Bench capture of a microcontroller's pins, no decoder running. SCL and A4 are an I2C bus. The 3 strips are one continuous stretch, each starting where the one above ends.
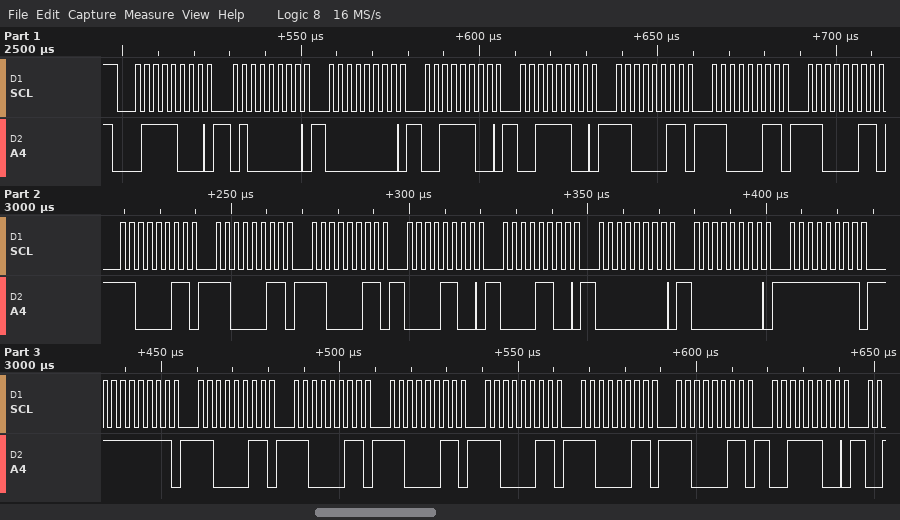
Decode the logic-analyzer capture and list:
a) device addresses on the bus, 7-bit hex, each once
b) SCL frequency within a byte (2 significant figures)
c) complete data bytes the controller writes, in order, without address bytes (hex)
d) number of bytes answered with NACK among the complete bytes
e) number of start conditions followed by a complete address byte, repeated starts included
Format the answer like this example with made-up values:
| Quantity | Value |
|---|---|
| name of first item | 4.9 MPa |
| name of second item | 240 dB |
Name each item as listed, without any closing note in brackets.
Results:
| Quantity | Value |
|---|---|
| device addresses on the bus, 7-bit hex, each once | 0x3C |
| SCL frequency within a byte | 400 kHz |
| complete data bytes the controller writes, in order, without address bytes | 40 00 3C 3C C3 C3 C3 C3 C3 C3 0C 0C 00 00 FF FF C3 C3 C3 C3 C3 C3 3C |
| number of bytes answered with NACK among the complete bytes | 0 |
| number of start conditions followed by a complete address byte, repeated starts included | 1 |
